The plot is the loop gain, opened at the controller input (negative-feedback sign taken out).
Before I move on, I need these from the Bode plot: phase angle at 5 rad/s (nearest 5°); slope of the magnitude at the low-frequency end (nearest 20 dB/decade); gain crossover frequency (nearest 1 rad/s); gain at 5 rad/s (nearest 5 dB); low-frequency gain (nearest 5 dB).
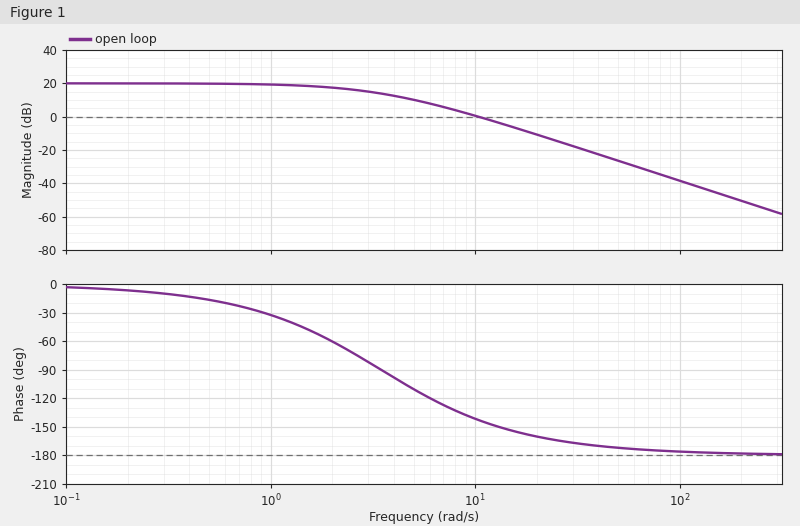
-110°
0 dB/decade
10 rad/s
10 dB
20 dB
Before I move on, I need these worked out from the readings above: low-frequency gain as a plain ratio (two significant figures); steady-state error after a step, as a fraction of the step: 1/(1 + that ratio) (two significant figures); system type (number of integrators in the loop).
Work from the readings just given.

10
0.091
0
